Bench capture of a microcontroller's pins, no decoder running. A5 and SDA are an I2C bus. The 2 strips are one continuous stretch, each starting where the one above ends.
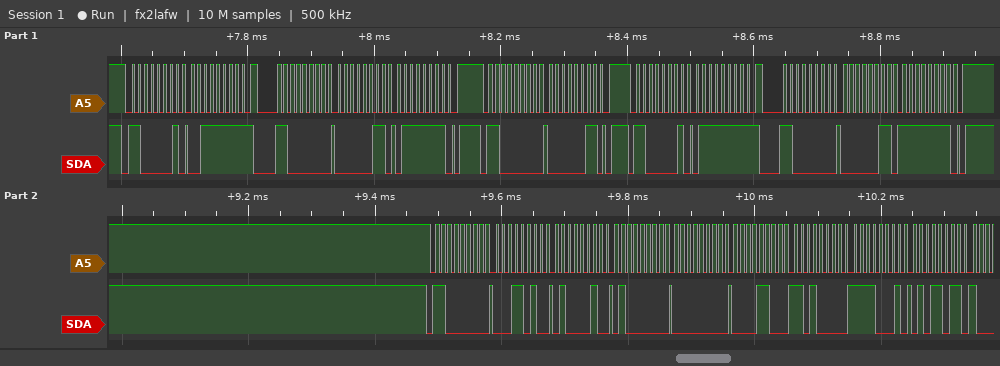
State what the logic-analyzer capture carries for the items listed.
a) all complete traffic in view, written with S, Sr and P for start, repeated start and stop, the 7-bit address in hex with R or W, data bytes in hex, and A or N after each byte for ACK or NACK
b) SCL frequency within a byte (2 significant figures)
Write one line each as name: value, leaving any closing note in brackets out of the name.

all complete traffic in view, written with S, Sr and P for start, repeated start and stop, the 7-bit address in hex with R or W, data bytes in hex, and A or N after each byte for ACK or NACK: S 60R A 3F N Sr 60W A 03 A 7F A P S 60W A 03 A P S 60R A 7F N Sr 60W A 03 A FF A P S 60W A 1A A 42 A 40 A 00 A 0C A D0 A F1 A 5B A
SCL frequency within a byte: 100 kHz
